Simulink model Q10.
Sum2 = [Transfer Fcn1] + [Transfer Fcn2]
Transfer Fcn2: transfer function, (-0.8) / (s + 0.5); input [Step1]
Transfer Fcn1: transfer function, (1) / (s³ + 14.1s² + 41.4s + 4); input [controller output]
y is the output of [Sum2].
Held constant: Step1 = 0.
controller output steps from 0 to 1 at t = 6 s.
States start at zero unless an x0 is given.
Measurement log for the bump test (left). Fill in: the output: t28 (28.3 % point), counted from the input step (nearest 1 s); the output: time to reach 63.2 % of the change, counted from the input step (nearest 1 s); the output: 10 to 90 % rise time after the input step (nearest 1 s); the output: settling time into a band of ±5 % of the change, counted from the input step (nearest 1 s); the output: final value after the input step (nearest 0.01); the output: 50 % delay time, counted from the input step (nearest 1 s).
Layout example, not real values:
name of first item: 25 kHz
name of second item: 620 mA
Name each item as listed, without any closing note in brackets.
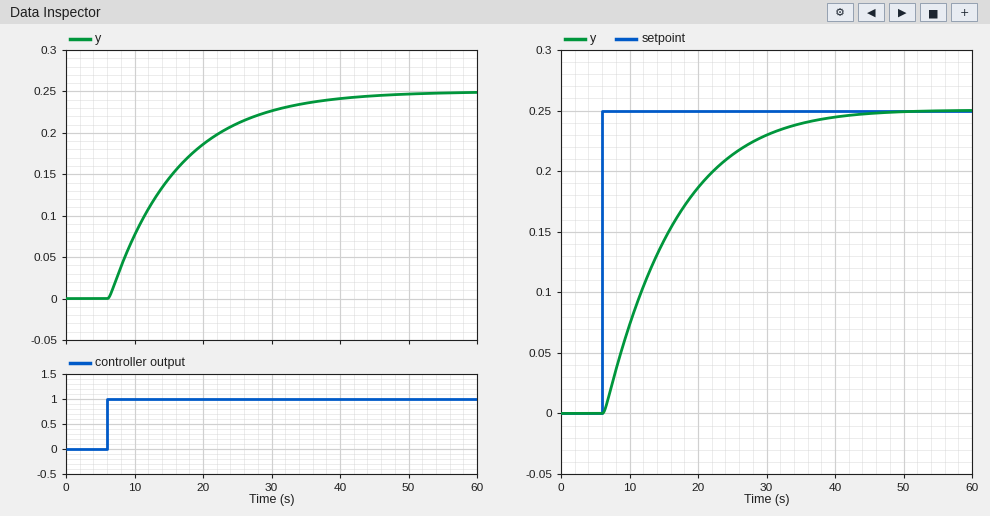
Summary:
the output: t28 (28.3 % point), counted from the input step: 4 s
the output: time to reach 63.2 % of the change, counted from the input step: 10 s
the output: 10 to 90 % rise time after the input step: 22 s
the output: settling time into a band of ±5 % of the change, counted from the input step: 30 s
the output: final value after the input step: 0.25
the output: 50 % delay time, counted from the input step: 7 s
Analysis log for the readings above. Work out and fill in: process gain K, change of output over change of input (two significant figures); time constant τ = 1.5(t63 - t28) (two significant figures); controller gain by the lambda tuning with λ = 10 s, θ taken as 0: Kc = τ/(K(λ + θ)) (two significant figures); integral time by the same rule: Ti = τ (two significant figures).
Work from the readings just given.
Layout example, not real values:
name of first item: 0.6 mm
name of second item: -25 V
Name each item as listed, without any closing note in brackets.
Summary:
process gain K, change of output over change of input: 0.25
time constant τ = 1.5(t63 - t28): 9.0 s
controller gain by the lambda tuning with λ = 10 s, θ taken as 0: Kc = τ/(K(λ + θ)): 3.6
integral time by the same rule: Ti = τ: 9.0 s
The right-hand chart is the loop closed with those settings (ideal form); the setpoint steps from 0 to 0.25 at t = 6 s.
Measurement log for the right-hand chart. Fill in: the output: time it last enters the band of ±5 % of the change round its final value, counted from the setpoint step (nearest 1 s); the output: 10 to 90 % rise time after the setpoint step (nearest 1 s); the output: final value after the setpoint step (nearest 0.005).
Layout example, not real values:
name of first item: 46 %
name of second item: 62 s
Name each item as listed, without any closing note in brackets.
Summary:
the output: time it last enters the band of ±5 % of the change round its final value, counted from the setpoint step: 28 s
the output: 10 to 90 % rise time after the setpoint step: 21 s
the output: final value after the setpoint step: 0.250
